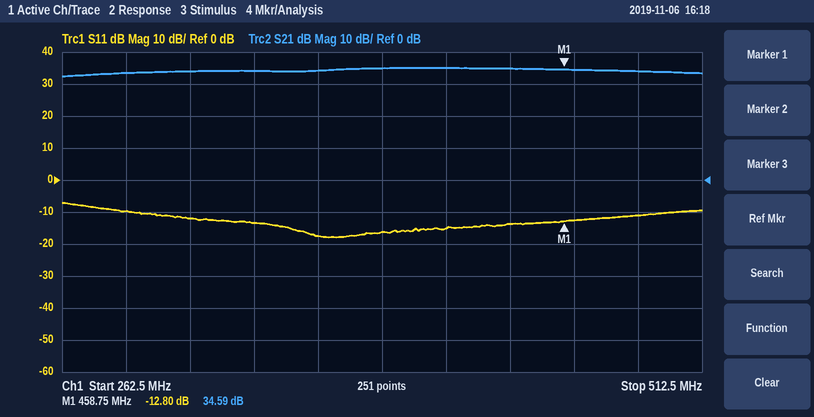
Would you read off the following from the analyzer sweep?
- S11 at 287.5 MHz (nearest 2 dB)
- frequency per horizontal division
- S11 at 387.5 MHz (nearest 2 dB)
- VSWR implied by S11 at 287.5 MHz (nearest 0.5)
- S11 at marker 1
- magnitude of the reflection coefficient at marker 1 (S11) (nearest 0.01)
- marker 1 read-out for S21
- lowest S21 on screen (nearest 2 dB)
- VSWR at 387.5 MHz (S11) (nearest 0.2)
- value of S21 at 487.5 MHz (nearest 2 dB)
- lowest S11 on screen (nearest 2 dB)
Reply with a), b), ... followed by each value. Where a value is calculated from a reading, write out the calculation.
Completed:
a) -10 dB
b) 25 MHz
c) -16 dB
d) |Γ| = 10^(-10/20) = 0.3162; VSWR = (1 + 0.3162)/(1 − 0.3162) ≈ 1.92, so 2.0 to the nearest 0.5
e) -12.80 dB
f) 10^(-12.8/20) ≈ 0.23
g) 34.59 dB
h) 32 dB
i) |Γ| = 10^(-16/20) = 0.1585; VSWR = (1 + 0.1585)/(1 − 0.1585) ≈ 1.4
j) 34 dB
k) -18 dB
